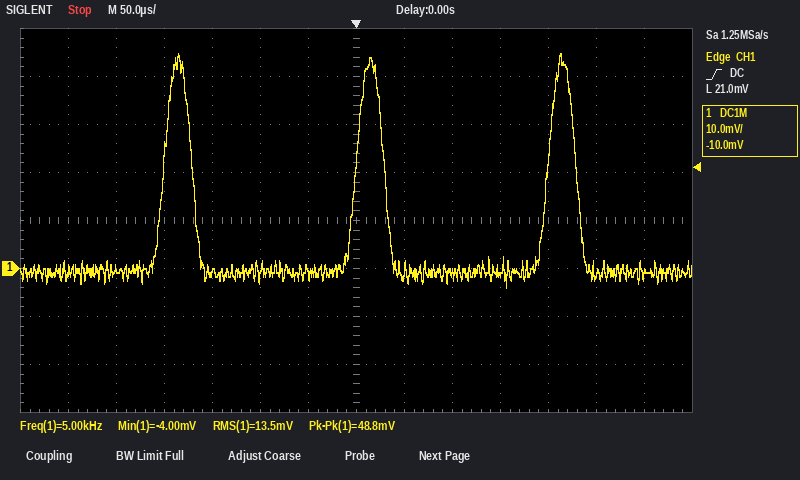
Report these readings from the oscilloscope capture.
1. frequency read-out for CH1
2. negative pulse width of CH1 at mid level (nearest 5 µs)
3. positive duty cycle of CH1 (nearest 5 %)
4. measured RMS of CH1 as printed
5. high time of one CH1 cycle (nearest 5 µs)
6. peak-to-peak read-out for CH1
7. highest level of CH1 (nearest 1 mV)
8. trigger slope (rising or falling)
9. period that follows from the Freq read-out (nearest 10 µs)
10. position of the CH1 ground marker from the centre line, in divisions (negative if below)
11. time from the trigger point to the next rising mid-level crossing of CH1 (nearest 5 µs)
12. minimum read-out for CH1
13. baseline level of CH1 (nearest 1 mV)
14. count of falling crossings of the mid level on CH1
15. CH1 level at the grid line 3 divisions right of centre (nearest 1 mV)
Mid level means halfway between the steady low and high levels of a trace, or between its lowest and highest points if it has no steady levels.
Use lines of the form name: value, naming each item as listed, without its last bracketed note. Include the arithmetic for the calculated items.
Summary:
frequency read-out for CH1: 5.00 kHz
negative pulse width of CH1 at mid level: 170 µs
positive duty cycle of CH1: 15 %
measured RMS of CH1 as printed: 13.5 mV
high time of one CH1 cycle: 30 µs
peak-to-peak read-out for CH1: 48.8 mV
highest level of CH1: 45 mV
trigger slope: rising
period that follows from the Freq read-out: 1 / 5.00 kHz ≈ 200 µs
position of the CH1 ground marker from the centre line, in divisions: -1.0 div
time from the trigger point to the next rising mid-level crossing of CH1: 200 µs
minimum read-out for CH1: -4.00 mV
baseline level of CH1: -1 mV
count of falling crossings of the mid level on CH1: 3
CH1 level at the grid line 3 divisions right of centre: -1 mV
